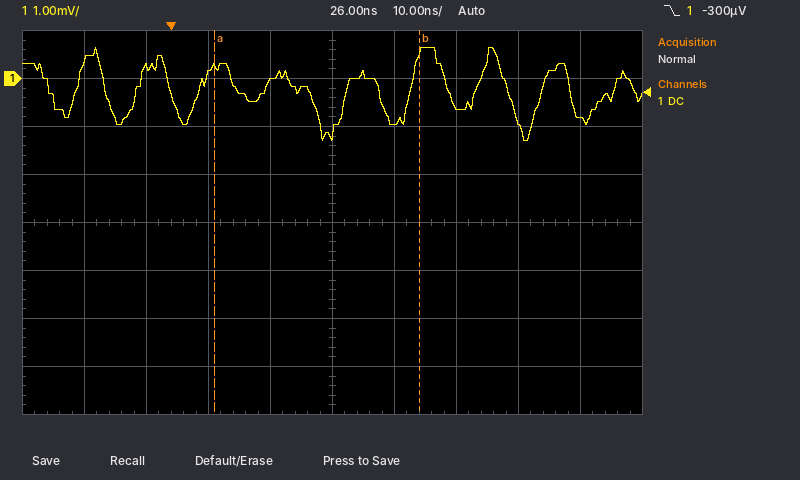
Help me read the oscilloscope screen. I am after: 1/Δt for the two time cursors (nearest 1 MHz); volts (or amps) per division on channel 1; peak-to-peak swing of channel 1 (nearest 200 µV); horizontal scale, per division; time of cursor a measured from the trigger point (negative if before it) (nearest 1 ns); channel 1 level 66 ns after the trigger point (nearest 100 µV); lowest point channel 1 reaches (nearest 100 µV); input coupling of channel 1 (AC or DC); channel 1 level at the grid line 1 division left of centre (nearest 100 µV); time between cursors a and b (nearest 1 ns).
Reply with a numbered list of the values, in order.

1. 30 MHz
2. 1 mV
3. 2.0 mV
4. 10 ns
5. +7 ns
6. -800 µV
7. -1.3 mV
8. DC
9. -100 µV
10. 33 ns
